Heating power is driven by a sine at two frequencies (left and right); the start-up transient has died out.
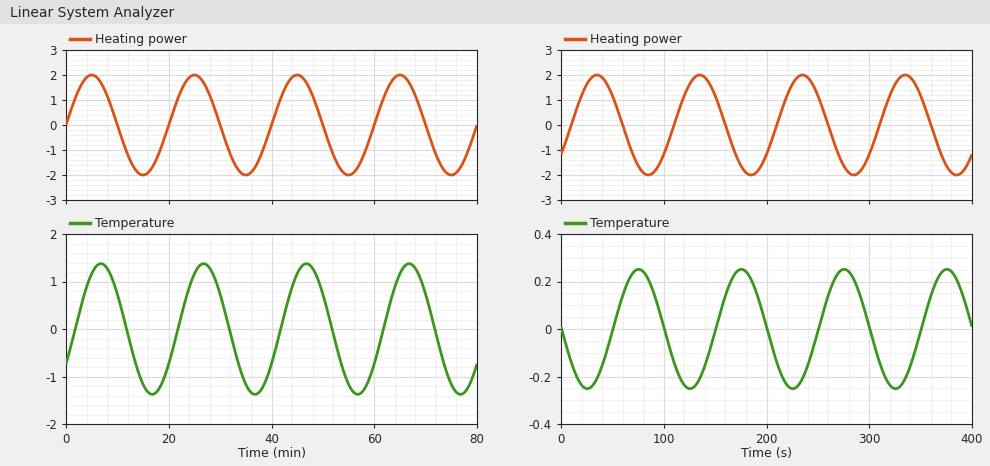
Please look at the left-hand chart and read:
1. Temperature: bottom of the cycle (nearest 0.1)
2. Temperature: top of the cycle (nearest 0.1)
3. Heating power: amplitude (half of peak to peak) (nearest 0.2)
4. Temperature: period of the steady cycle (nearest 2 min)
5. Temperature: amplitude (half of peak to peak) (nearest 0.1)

-1.4
1.4
2.0
20 min
1.4
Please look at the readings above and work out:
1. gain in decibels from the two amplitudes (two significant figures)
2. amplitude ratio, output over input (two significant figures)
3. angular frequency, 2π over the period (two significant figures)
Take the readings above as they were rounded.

-3.1 dB
0.70
0.31 rad/min
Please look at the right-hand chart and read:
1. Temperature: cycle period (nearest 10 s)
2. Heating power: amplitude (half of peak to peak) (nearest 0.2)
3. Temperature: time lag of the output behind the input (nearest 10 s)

100 s
2.0
40 s
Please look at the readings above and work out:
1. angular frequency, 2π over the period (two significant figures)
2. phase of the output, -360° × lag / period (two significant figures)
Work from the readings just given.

0.063 rad/s
-140°
